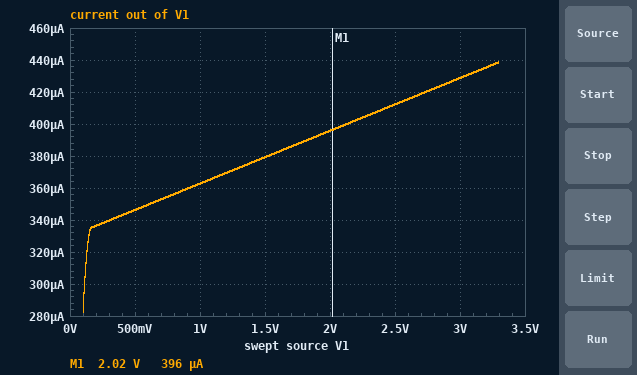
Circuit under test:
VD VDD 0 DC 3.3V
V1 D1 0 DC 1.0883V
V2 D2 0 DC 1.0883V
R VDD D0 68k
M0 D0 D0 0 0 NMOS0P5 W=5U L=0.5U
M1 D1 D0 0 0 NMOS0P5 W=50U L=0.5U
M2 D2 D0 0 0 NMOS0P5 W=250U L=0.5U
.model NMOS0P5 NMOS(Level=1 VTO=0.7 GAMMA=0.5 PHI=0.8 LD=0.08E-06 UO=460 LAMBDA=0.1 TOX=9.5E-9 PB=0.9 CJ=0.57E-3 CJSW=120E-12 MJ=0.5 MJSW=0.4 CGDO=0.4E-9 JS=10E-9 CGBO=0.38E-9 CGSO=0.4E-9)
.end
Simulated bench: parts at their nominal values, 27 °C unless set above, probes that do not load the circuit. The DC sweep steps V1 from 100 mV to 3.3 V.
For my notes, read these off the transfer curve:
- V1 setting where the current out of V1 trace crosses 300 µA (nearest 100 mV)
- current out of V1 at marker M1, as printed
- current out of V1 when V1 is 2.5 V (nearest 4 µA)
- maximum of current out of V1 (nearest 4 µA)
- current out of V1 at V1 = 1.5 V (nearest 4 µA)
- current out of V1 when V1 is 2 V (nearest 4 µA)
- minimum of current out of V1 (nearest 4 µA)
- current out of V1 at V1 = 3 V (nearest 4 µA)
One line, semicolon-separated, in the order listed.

100 mV; 396 µA; 412 µA; 440 µA; 380 µA; 396 µA; 284 µA; 428 µA
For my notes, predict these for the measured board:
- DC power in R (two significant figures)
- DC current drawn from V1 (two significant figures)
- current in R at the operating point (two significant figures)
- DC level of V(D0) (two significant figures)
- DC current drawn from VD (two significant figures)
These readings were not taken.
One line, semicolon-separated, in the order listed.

87 µW; 370 µA; 36 µA; 860 mV; 36 µA
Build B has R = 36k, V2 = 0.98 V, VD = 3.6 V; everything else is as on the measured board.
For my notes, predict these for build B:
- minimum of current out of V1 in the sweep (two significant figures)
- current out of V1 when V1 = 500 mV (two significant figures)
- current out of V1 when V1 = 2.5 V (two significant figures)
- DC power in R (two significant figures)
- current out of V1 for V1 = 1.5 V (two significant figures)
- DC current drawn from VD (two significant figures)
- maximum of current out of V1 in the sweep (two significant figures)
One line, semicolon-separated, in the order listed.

460 µA; 710 µA; 850 µA; 200 µW; 780 µA; 74 µA; 900 µA
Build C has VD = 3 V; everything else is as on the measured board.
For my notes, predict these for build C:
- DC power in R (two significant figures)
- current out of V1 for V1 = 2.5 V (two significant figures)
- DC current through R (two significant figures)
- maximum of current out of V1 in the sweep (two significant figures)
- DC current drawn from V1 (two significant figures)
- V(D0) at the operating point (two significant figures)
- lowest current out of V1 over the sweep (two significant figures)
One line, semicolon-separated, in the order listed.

68 µW; 360 µA; 32 µA; 390 µA; 320 µA; 850 mV; 260 µA
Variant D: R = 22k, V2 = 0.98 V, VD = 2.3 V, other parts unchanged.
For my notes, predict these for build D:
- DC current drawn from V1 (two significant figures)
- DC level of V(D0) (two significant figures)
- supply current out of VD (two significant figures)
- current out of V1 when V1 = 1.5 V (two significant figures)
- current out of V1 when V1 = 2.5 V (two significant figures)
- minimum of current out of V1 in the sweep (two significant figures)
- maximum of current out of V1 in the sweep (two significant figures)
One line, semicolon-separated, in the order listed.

640 µA; 920 mV; 63 µA; 660 µA; 720 µA; 410 µA; 770 µA
